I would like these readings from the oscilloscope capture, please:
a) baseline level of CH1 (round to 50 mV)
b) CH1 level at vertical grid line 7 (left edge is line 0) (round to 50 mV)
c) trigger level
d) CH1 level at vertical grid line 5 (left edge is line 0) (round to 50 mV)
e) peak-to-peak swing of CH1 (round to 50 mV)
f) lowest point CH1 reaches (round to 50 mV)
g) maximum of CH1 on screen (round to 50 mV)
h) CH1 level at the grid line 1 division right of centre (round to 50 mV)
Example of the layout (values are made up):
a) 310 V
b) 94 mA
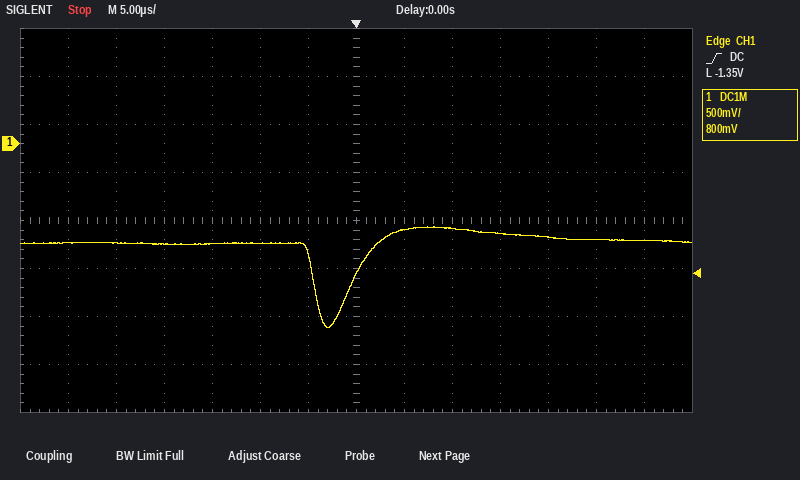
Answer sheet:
a) -1.05 V
b) -1.35 V
c) -1.35 V
d) -1.05 V
e) 1.05 V
f) -1.90 V
g) -850 mV
h) -900 mV
